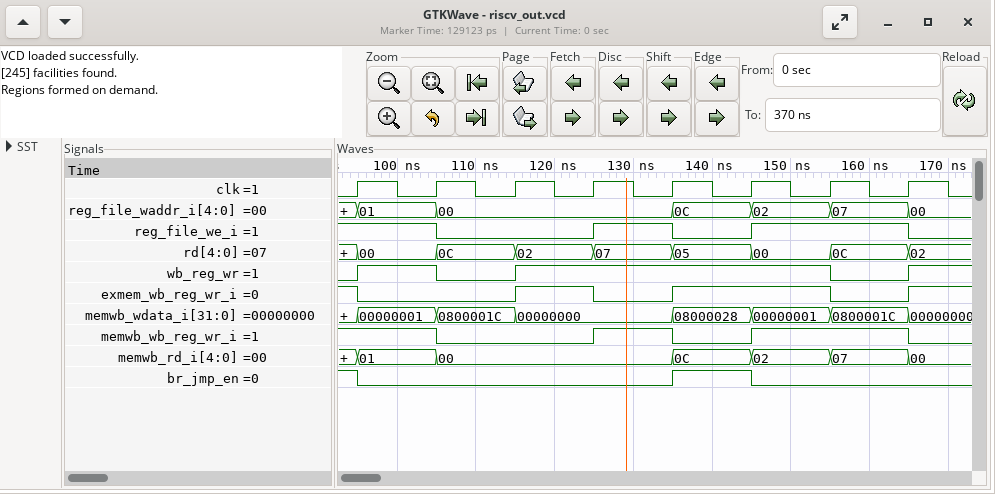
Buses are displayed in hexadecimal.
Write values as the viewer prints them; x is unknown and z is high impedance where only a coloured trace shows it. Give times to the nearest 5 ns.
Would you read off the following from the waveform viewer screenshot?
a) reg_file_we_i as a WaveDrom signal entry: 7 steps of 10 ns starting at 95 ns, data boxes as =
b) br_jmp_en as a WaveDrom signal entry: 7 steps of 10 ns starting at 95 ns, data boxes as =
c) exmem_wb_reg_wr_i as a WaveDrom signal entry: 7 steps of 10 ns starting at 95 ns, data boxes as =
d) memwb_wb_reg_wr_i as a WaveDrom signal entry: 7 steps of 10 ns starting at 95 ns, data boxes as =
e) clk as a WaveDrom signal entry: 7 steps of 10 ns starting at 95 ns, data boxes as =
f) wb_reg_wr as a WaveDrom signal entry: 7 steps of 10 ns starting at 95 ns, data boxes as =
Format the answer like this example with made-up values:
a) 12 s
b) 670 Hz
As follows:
a) {name: 'reg_file_we_i', wave: '10.101.'}
b) {name: 'br_jmp_en', wave: '0...10.'}
c) {name: 'exmem_wb_reg_wr_i', wave: '0.101.0'}
d) {name: 'memwb_wb_reg_wr_i', wave: '10.101.'}
e) {name: 'clk', wave: 'p......'}
f) {name: 'wb_reg_wr', wave: '101...0'}
